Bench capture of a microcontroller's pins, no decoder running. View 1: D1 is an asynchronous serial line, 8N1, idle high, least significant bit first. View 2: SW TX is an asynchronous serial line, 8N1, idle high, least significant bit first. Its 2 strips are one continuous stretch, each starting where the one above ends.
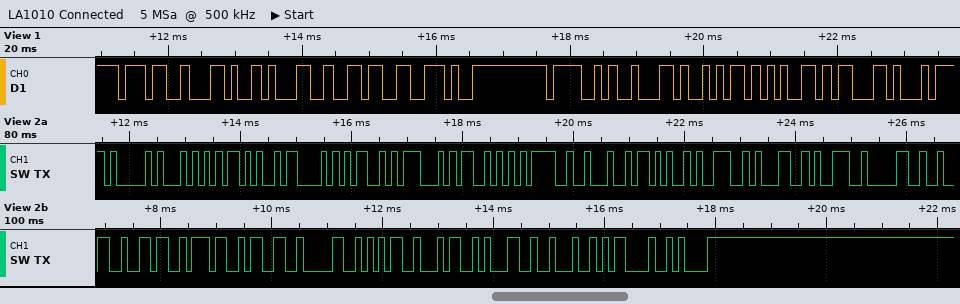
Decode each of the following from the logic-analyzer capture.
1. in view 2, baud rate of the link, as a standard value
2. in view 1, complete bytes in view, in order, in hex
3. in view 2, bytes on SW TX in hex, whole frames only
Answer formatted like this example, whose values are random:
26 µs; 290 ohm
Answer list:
9600 baud; 37 2C 31 36 2E 4F 62 6A 65 63; 41 54 2B 43 4D 47 53 3D 22 2B 39 31 39 30 32 36 37 33 30 35 34 31 22 0D 0A
